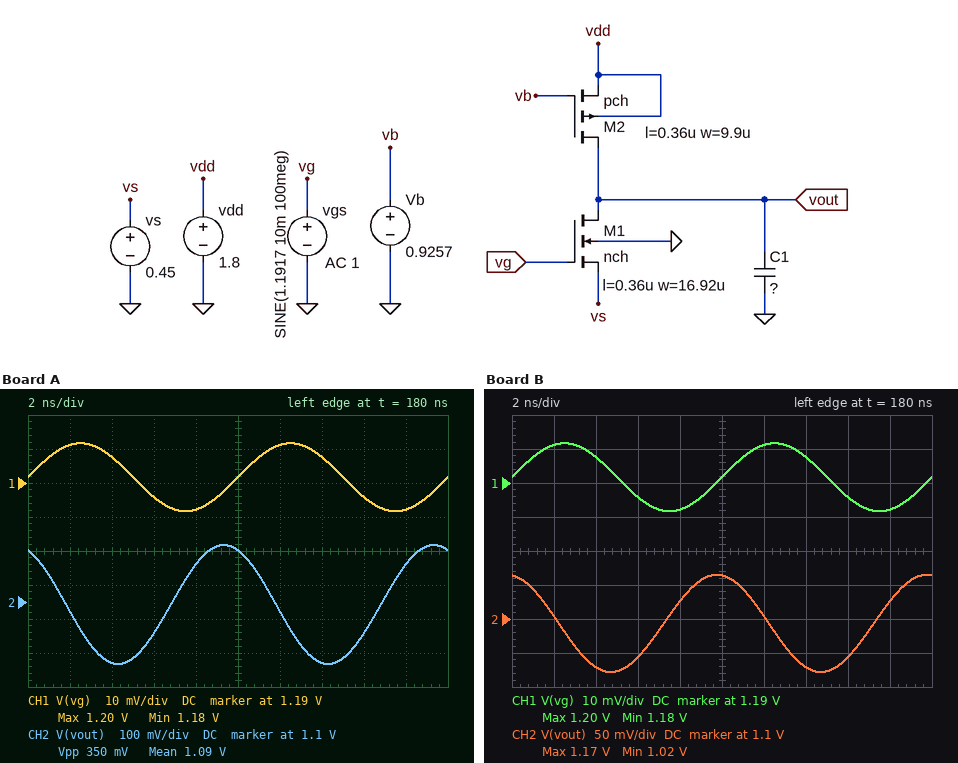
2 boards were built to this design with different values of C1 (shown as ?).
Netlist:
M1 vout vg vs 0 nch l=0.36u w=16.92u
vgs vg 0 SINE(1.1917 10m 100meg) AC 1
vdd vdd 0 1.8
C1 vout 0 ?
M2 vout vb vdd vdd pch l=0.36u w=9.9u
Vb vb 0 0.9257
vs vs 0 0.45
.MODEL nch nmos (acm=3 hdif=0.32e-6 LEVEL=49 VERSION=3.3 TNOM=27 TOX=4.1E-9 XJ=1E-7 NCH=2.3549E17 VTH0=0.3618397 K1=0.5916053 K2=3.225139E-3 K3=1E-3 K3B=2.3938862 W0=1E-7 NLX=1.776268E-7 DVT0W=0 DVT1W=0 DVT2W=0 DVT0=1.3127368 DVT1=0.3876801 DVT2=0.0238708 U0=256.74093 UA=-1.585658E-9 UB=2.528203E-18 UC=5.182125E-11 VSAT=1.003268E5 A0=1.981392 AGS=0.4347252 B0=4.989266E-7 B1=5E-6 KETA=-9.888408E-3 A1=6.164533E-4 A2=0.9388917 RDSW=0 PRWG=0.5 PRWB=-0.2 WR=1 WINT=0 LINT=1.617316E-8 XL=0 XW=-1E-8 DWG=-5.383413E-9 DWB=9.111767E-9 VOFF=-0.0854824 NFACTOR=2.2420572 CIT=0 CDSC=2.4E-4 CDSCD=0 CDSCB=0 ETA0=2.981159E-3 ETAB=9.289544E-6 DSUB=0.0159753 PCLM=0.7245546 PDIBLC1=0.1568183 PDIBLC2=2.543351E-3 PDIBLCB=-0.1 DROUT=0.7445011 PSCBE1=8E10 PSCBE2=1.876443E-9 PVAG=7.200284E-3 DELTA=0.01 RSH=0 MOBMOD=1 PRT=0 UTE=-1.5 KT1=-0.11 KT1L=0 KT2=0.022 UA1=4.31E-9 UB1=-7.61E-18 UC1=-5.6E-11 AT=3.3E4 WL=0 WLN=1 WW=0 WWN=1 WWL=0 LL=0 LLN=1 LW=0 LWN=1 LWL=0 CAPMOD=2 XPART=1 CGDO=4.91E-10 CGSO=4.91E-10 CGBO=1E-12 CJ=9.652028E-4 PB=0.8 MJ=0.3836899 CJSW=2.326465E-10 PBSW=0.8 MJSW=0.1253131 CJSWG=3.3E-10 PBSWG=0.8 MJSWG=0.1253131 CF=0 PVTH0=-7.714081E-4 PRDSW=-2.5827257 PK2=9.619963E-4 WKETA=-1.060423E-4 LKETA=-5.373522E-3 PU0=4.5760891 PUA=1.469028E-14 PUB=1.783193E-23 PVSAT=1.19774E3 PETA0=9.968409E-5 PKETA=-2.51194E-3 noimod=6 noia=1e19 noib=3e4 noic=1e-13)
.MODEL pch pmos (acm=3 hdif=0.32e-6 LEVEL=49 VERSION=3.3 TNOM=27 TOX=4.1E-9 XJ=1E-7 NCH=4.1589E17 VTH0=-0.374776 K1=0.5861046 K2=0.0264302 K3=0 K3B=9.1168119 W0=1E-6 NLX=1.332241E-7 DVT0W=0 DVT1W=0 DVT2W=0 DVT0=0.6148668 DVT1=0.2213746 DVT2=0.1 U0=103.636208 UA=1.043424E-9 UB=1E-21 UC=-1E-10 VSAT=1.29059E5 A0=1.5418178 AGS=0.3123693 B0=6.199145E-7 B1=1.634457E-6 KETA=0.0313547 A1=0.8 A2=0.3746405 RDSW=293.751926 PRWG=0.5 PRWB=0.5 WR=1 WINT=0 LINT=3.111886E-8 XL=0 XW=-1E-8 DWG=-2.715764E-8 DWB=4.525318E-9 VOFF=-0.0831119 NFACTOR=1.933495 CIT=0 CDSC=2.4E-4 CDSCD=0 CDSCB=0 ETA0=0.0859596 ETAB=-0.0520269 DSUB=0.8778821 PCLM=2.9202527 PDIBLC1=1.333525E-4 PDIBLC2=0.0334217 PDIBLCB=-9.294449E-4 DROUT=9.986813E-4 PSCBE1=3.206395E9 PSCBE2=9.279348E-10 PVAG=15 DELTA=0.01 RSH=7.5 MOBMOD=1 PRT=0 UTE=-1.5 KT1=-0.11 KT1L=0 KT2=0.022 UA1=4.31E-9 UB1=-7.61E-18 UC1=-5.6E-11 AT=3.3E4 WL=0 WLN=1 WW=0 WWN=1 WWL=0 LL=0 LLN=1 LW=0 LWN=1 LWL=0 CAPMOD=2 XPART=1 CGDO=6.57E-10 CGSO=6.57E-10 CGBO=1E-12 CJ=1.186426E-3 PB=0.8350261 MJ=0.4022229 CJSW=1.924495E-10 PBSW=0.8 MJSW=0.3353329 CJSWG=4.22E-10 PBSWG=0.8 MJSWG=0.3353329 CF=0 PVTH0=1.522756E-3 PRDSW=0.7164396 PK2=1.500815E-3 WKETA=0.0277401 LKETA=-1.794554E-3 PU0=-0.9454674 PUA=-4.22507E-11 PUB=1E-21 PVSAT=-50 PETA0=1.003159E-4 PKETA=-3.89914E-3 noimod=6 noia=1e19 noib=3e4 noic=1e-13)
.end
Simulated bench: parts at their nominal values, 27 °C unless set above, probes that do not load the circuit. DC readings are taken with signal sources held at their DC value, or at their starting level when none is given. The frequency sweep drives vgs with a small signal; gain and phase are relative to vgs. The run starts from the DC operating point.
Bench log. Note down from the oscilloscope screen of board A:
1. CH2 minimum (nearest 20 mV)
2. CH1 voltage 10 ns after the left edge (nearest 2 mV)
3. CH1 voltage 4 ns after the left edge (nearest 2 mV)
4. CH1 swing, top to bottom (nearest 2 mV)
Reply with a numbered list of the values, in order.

1. 920 mV
2. 1.192 V
3. 1.198 V
4. 20 mV
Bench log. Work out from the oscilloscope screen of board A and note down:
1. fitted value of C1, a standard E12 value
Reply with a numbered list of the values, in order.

1. 120 fF
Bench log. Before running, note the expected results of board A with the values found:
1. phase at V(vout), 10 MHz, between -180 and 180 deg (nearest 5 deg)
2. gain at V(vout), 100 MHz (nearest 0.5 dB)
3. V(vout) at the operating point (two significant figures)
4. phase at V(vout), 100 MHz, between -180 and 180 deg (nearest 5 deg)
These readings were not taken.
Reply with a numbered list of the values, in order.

1. 170 deg
2. 25.0 dB
3. 1.1 V
4. 115 deg
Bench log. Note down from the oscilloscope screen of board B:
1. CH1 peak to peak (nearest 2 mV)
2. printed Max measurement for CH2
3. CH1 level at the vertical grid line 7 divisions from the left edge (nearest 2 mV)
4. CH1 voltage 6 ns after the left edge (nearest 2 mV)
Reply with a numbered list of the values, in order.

1. 20 mV
2. 1.17 V
3. 1.198 V
4. 1.186 V
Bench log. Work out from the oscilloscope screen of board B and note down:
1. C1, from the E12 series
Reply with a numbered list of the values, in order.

1. 390 fF
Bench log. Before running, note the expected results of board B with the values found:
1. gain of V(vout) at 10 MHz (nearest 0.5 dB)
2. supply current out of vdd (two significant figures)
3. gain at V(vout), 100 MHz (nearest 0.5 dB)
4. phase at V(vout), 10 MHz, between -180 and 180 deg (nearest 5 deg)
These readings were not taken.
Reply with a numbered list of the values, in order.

1. 31.0 dB
2. 170 µA
3. 17.0 dB
4. 150 deg
